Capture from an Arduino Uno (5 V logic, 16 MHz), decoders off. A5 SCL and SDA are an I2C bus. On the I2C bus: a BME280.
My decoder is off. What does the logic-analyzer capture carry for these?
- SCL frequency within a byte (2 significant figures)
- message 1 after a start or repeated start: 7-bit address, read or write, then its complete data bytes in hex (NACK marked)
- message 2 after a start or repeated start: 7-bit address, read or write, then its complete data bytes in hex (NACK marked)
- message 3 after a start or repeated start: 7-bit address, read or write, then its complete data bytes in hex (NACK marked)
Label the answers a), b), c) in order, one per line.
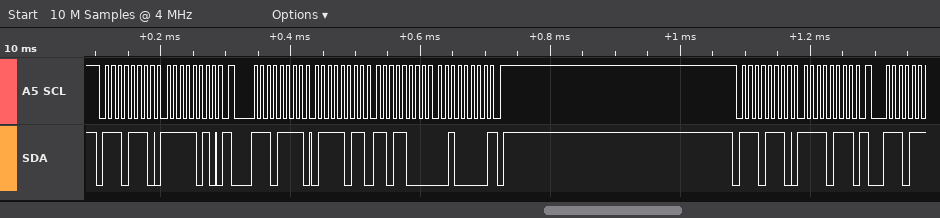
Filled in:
a) 100 kHz
b) 0x77 write: FA
c) 0x77 read: 7B D8 20 NACK
d) 0x77 write: F7
